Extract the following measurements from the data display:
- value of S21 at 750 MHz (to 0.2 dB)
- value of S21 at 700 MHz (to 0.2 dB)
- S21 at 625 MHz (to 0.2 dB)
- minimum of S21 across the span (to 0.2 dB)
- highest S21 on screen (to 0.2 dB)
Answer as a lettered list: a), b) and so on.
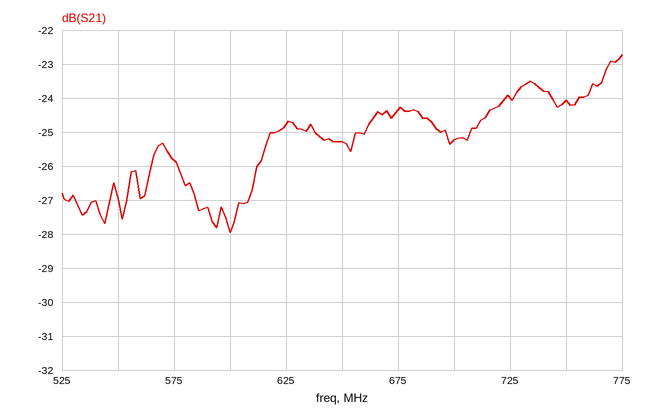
a) -24.0 dB
b) -25.2 dB
c) -24.8 dB
d) -28.0 dB
e) -22.8 dB
